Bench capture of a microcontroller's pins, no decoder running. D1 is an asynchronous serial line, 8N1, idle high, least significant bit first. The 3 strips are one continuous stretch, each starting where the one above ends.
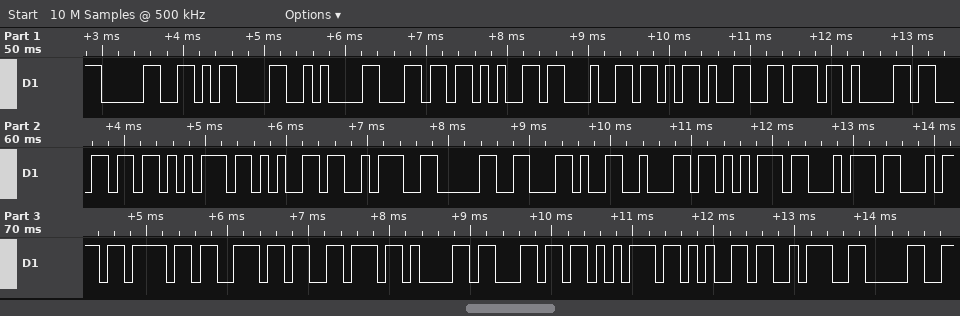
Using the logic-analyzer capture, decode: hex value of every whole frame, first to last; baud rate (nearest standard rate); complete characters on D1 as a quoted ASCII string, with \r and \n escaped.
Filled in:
30 0D 0A 6C 65 64 2D 76 61 6C 75 65 3A 30 2C 62 75 74 74 6F 6E 76 61 6C 75 65 3A 30
9600 baud
"0\r\nled-value:0,buttonvalue:0"
